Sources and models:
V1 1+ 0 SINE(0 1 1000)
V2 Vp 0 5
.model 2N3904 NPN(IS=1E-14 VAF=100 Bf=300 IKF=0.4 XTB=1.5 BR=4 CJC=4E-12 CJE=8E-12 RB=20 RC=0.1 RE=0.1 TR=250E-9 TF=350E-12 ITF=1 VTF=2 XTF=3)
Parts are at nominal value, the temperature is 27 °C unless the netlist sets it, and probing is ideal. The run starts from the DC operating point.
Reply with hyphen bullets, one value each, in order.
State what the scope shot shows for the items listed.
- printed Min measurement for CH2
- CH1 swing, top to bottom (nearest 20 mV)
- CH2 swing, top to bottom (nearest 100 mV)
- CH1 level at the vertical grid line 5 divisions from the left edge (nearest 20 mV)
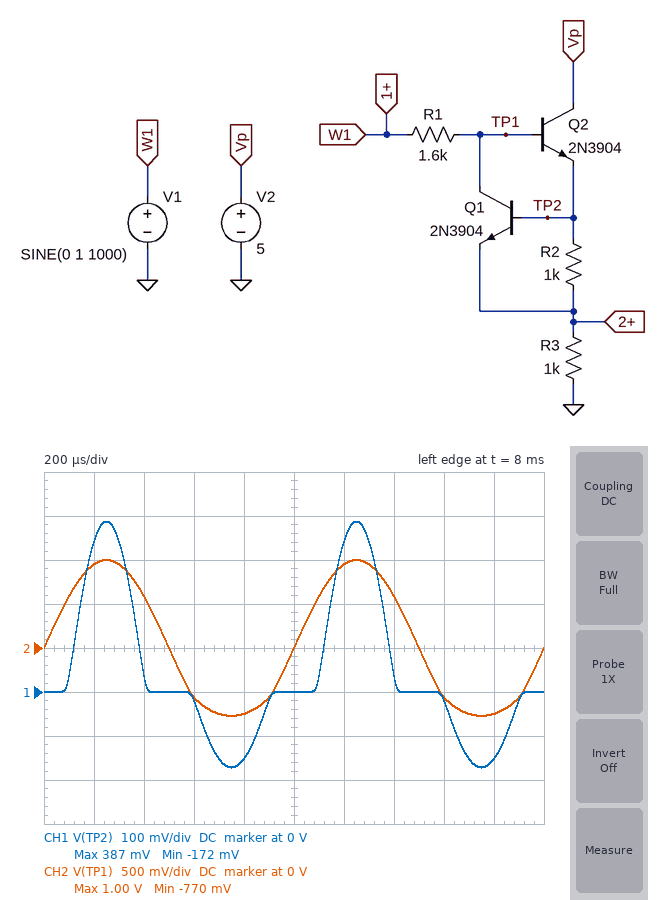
- -770 mV
- 560 mV
- 1.8 V
- 0 V
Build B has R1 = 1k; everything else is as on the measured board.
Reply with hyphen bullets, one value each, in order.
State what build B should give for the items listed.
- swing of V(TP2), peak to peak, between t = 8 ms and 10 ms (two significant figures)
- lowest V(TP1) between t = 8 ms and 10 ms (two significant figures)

- 600 mV
- -820 mV
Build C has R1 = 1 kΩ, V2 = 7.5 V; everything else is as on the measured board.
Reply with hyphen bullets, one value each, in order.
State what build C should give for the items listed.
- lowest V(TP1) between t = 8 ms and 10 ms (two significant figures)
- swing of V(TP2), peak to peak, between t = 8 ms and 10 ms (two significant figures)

- -820 mV
- 600 mV
